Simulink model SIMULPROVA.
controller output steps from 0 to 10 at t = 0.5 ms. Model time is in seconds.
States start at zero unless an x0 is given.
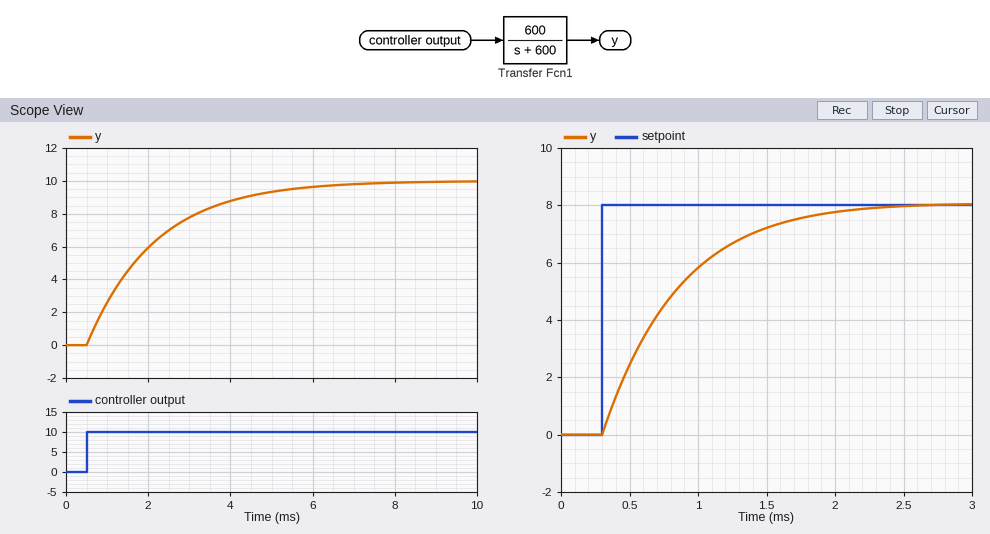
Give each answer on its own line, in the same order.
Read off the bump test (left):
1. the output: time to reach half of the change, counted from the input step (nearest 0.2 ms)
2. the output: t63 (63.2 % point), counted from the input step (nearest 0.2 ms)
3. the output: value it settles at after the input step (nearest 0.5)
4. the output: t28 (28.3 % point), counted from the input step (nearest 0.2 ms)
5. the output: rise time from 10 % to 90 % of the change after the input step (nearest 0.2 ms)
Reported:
1.2 ms
1.6 ms
10.0
0.6 ms
3.6 ms
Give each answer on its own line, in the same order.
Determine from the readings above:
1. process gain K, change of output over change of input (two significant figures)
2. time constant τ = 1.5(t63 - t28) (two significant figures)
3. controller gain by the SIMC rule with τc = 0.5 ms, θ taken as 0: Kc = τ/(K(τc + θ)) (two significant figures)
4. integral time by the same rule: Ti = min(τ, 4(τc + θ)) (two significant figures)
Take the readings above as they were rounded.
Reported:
1.0
1.5 ms
3.0
1.5 ms
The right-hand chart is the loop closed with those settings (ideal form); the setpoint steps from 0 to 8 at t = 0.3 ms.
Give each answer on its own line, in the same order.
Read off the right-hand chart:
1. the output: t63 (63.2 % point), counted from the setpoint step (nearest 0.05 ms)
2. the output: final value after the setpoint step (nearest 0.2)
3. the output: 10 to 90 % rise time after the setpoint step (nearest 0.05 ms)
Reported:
0.55 ms
8.0
1.15 ms
